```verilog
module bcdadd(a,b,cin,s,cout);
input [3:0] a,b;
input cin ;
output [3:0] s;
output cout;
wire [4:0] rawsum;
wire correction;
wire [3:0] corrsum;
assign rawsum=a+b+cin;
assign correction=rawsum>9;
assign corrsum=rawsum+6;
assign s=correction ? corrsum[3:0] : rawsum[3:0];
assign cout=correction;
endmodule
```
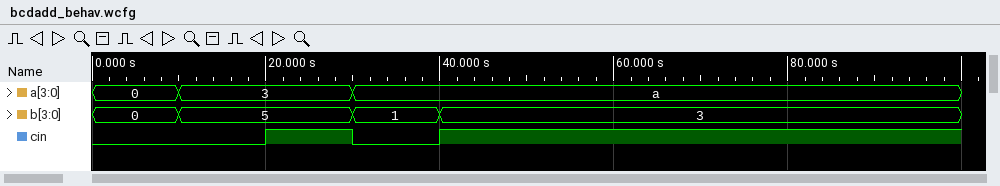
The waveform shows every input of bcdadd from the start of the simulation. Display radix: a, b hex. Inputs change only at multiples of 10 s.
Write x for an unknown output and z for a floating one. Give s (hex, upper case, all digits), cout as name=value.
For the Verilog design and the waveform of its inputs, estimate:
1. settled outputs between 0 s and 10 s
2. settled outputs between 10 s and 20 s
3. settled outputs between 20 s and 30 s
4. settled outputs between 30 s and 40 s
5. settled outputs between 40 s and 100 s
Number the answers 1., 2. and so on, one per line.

1. s=0, cout=0
2. s=8, cout=0
3. s=9, cout=0
4. s=1, cout=1
5. s=4, cout=1
